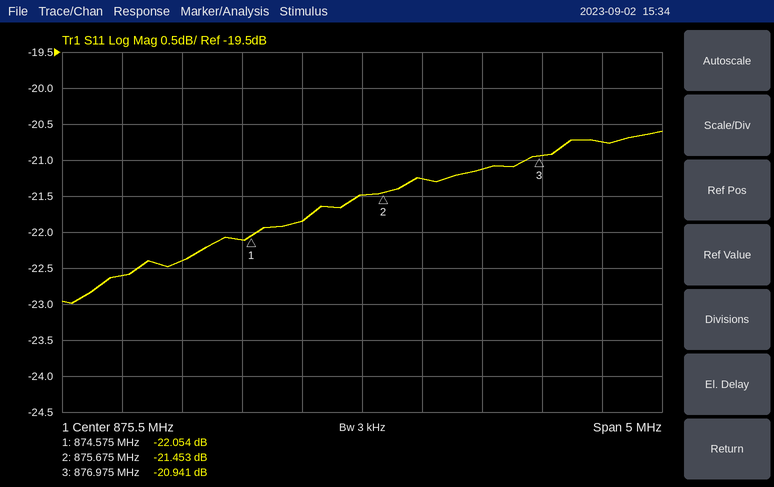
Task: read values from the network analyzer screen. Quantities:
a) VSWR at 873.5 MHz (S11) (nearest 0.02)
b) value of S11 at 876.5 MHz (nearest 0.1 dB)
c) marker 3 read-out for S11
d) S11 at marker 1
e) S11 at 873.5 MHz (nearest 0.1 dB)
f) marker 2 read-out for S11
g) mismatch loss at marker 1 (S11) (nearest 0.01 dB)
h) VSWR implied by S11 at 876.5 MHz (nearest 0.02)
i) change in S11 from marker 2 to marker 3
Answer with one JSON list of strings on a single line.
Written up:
["1.16", "-21.1 dB", "-20.941 dB", "-22.054 dB", "-22.6 dB", "-21.453 dB", "0.03 dB", "1.20", "0.512 dB"]
